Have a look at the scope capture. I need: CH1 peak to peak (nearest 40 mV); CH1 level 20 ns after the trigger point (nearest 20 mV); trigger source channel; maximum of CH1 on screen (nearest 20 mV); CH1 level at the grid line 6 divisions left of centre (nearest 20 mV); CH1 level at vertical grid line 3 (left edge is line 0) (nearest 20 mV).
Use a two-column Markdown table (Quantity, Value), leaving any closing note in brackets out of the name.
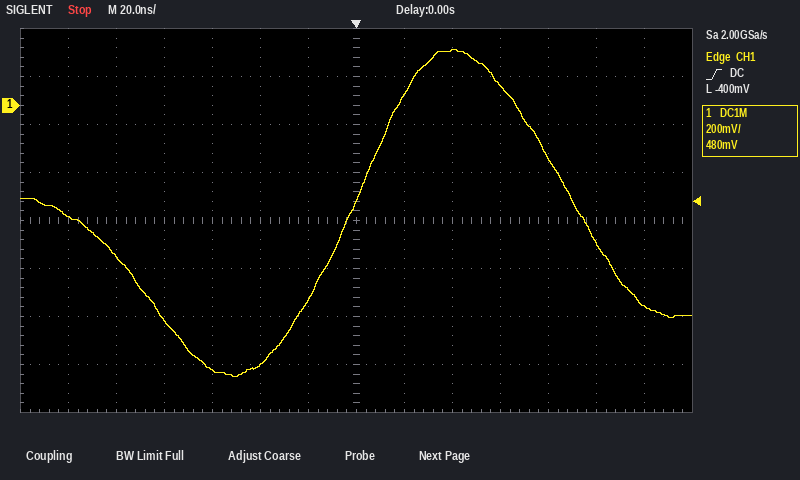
| Quantity | Value |
|---|---|
| CH1 peak to peak | 1.36 V |
| CH1 level 20 ns after the trigger point | 40 mV |
| trigger source channel | CH1 |
| maximum of CH1 on screen | 240 mV |
| CH1 level at the grid line 6 divisions left of centre | -460 mV |
| CH1 level at vertical grid line 3 (left edge is line 0) | -900 mV |
